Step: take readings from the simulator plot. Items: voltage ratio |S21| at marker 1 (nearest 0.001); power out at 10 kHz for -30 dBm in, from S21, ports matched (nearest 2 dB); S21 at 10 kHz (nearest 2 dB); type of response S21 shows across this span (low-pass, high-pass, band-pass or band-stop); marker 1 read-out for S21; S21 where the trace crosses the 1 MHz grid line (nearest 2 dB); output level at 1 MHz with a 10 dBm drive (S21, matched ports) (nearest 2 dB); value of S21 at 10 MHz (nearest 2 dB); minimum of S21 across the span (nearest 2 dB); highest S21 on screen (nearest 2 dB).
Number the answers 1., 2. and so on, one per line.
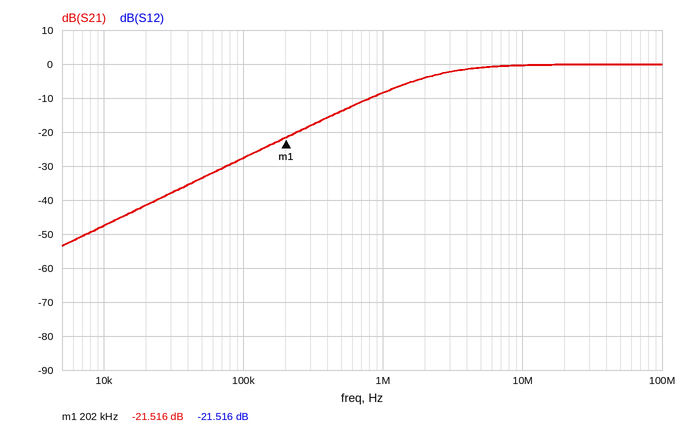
1. 0.084
2. -78 dBm
3. -48 dB
4. high-pass
5. -21.516 dB
6. -8 dB
7. 2 dBm
8. 0 dB
9. -54 dB
10. 0 dB
